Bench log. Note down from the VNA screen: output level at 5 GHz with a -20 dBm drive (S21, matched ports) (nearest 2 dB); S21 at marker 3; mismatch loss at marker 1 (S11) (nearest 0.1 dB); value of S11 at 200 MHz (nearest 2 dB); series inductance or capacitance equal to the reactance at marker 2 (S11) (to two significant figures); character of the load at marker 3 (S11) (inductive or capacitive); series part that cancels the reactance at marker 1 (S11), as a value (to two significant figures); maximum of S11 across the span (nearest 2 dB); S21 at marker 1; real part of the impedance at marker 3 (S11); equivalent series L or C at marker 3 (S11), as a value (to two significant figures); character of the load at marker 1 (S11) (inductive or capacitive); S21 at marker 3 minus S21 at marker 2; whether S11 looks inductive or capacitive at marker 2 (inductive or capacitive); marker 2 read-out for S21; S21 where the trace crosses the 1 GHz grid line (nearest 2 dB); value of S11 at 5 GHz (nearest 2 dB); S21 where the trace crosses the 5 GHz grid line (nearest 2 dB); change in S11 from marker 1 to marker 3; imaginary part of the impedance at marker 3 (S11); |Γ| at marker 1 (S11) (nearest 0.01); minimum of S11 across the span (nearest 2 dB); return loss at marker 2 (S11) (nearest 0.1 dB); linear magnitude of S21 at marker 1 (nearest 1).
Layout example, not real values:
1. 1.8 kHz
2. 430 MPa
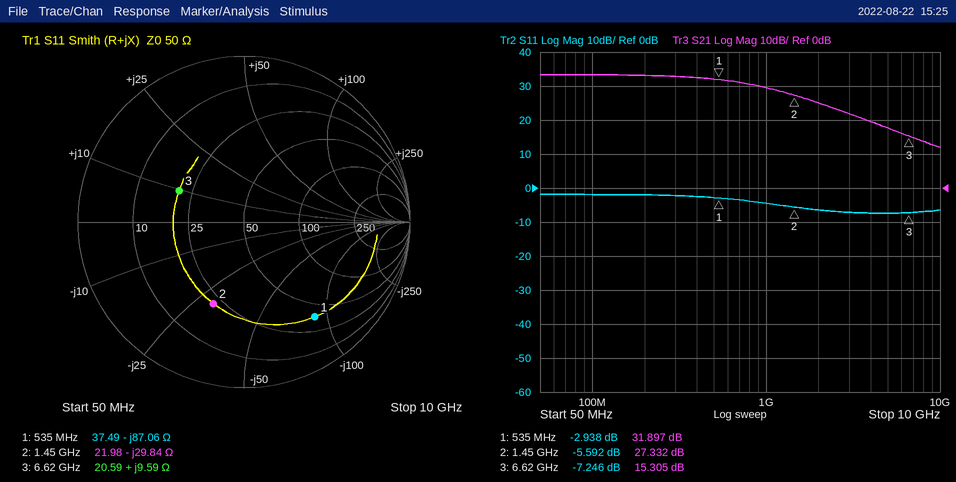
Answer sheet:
1. -2 dBm
2. 15.305 dB
3. 3.1 dB
4. -2 dB
5. 3.7 pF
6. inductive
7. 26 nH
8. -2 dB
9. 31.897 dB
10. 20.59 Ω
11. 230 pH
12. capacitive
13. -12.027 dB
14. capacitive
15. 27.332 dB
16. 30 dB
17. -8 dB
18. 18 dB
19. -4.308 dB
20. +9.59 Ω
21. 0.71
22. -8 dB
23. 5.6 dB
24. 39
